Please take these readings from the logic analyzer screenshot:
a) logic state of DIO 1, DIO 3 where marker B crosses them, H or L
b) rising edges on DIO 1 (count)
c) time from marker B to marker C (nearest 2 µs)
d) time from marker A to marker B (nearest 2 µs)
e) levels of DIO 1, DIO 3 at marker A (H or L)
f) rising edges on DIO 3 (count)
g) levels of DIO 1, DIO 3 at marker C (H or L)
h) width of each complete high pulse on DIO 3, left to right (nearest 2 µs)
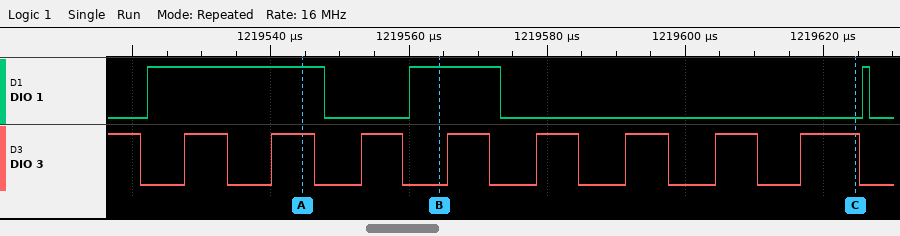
DIO 1=H, DIO 3=L
3
60 µs
20 µs
DIO 1=H, DIO 3=H
8
DIO 1=L, DIO 3=H
6 µs, 6 µs, 6 µs, 6 µs, 6 µs, 6 µs, 6 µs, 8 µs
